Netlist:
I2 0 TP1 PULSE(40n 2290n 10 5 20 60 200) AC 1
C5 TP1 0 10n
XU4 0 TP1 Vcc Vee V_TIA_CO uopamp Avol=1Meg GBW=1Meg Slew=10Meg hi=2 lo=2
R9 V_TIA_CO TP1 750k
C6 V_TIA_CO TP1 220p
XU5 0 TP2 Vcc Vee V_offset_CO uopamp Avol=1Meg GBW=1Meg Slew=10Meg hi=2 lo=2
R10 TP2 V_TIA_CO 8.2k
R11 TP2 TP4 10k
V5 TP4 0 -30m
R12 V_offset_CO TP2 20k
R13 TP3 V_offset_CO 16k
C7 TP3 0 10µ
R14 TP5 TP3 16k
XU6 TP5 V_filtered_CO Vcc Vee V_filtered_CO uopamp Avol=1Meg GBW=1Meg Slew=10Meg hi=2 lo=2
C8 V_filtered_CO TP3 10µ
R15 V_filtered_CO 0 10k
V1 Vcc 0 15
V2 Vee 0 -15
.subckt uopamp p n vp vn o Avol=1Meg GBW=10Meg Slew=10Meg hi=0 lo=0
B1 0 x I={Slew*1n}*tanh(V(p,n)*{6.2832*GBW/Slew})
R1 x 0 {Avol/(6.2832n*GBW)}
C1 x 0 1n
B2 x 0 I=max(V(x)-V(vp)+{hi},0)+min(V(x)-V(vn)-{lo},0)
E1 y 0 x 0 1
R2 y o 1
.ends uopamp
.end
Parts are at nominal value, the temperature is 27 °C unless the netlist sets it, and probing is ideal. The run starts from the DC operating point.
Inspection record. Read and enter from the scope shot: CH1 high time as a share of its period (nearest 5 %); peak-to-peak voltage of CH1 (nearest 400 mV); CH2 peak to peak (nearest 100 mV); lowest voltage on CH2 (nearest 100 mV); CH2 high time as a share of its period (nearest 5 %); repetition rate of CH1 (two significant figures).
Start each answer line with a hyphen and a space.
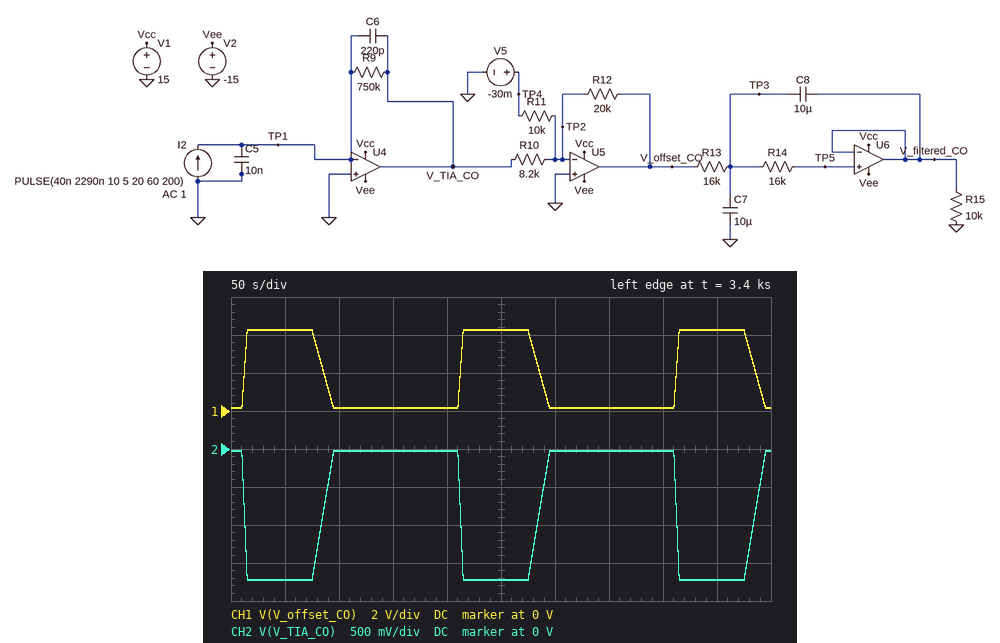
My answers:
- 35 %
- 4.0 V
- 1.7 V
- -1.7 V
- 65 %
- 5.0 mHz
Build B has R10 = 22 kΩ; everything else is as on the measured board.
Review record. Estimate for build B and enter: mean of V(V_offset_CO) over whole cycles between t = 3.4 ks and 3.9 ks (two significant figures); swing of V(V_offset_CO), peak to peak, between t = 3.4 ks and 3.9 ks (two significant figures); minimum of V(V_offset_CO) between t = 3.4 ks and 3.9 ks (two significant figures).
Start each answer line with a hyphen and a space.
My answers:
- 640 mV
- 1.5 V
- 87 mV
